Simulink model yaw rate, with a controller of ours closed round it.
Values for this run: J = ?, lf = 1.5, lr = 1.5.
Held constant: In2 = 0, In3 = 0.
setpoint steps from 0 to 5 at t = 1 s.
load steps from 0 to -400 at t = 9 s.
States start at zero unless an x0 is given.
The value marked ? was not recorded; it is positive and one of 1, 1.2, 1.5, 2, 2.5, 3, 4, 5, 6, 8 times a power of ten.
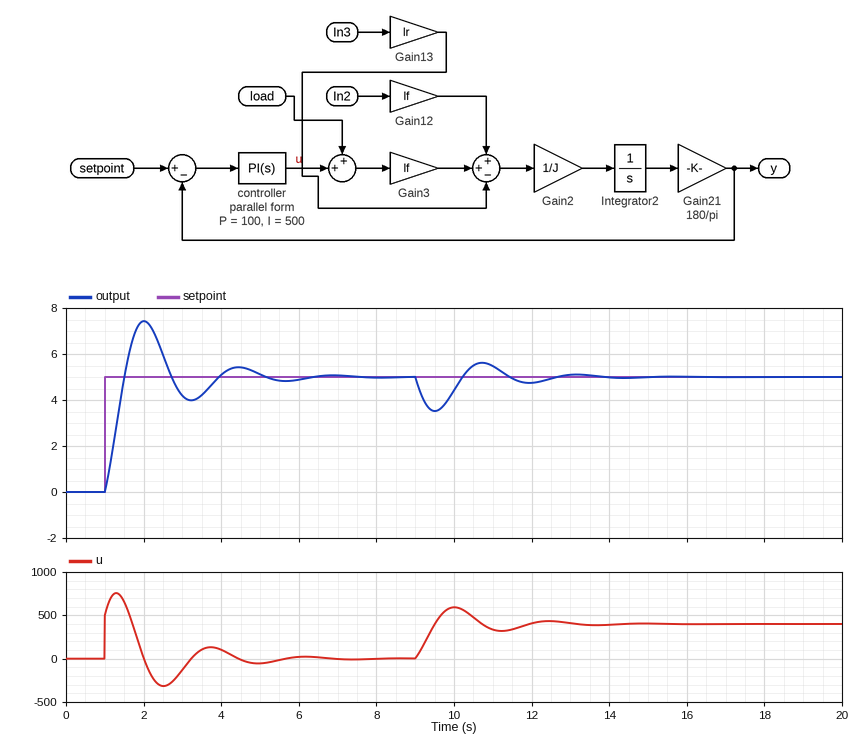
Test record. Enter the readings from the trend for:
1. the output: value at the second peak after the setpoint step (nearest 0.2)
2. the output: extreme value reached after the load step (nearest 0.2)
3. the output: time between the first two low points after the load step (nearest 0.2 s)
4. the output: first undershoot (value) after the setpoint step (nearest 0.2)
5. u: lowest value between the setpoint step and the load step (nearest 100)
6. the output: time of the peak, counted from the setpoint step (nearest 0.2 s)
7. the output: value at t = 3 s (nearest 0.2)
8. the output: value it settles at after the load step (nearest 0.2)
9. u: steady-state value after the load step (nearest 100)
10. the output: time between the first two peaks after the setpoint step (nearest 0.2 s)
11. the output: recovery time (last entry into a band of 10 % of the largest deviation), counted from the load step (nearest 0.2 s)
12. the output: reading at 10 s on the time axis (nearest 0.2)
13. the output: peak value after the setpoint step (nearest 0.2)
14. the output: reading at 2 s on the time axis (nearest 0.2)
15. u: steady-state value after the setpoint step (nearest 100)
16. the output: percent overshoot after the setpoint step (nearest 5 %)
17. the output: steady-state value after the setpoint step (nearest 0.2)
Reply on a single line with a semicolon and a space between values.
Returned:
5.4; 3.6; 2.4 s; 4.0; -300; 1.0 s; 4.2; 5.0; 400; 2.4 s; 3.4 s; 4.4; 7.4; 7.4; 0; 50 %; 5.0
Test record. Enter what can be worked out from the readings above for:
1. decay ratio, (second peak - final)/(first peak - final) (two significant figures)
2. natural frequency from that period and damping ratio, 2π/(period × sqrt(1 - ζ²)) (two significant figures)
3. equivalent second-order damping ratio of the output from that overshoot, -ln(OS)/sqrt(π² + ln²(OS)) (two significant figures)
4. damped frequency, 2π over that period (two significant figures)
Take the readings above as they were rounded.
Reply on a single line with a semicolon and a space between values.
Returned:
0.17; 2.7 rad/s; 0.22; 2.6 rad/s
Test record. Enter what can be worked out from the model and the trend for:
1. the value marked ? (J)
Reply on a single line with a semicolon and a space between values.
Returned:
6000
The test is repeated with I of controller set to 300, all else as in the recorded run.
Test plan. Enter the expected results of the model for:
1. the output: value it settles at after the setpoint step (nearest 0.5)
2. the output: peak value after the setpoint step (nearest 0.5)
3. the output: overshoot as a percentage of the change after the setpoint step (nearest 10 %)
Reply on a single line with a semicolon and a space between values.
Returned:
5.0; 7.0; 40 %
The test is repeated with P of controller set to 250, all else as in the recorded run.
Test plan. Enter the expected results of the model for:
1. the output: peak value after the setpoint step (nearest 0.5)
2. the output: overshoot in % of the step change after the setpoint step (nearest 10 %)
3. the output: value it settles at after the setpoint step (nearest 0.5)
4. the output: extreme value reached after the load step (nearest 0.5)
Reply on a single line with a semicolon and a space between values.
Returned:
6.0; 20 %; 5.0; 4.0
